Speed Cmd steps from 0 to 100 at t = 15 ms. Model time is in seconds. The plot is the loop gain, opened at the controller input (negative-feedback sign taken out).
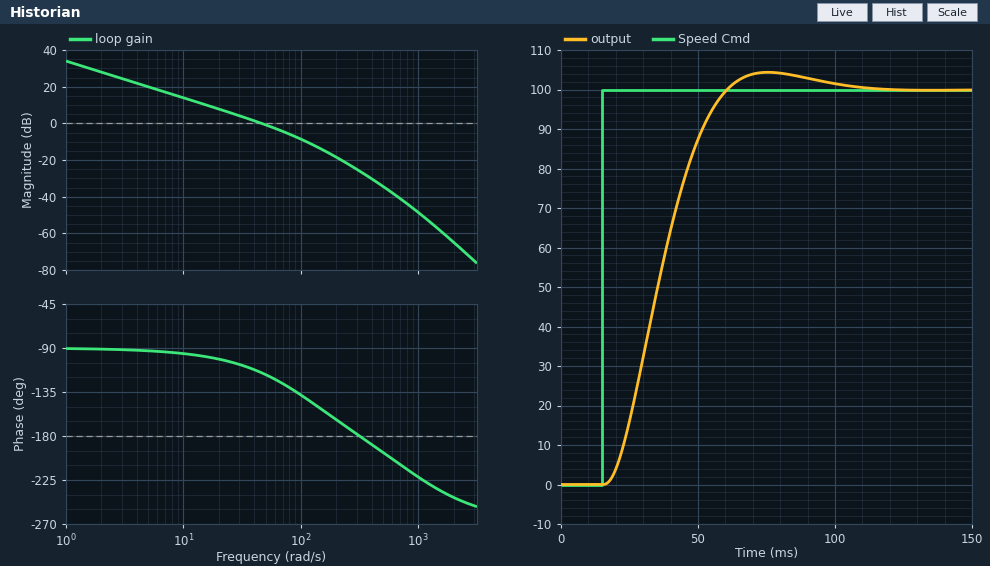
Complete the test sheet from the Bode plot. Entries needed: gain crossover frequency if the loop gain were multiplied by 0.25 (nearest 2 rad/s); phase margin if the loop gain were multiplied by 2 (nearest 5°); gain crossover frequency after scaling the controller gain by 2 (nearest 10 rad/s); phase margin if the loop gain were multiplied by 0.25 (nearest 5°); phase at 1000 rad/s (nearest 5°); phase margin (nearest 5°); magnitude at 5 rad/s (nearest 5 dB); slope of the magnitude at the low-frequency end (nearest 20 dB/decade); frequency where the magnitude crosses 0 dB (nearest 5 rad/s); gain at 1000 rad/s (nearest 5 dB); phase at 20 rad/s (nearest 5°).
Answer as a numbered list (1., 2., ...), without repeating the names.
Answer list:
1. 12 rad/s
2. 50°
3. 80 rad/s
4. 85°
5. -220°
6. 65°
7. 20 dB
8. -20 dB/decade
9. 45 rad/s
10. -50 dB
11. -100°
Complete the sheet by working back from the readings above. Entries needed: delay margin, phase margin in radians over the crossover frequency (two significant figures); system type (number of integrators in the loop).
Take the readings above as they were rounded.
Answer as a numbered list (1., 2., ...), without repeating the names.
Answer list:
1. 0.025 s
2. 1
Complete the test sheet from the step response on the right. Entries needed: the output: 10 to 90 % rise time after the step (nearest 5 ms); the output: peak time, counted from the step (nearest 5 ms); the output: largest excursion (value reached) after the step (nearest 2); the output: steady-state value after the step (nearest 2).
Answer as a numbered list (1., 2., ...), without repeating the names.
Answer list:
1. 30 ms
2. 60 ms
3. 104
4. 100
